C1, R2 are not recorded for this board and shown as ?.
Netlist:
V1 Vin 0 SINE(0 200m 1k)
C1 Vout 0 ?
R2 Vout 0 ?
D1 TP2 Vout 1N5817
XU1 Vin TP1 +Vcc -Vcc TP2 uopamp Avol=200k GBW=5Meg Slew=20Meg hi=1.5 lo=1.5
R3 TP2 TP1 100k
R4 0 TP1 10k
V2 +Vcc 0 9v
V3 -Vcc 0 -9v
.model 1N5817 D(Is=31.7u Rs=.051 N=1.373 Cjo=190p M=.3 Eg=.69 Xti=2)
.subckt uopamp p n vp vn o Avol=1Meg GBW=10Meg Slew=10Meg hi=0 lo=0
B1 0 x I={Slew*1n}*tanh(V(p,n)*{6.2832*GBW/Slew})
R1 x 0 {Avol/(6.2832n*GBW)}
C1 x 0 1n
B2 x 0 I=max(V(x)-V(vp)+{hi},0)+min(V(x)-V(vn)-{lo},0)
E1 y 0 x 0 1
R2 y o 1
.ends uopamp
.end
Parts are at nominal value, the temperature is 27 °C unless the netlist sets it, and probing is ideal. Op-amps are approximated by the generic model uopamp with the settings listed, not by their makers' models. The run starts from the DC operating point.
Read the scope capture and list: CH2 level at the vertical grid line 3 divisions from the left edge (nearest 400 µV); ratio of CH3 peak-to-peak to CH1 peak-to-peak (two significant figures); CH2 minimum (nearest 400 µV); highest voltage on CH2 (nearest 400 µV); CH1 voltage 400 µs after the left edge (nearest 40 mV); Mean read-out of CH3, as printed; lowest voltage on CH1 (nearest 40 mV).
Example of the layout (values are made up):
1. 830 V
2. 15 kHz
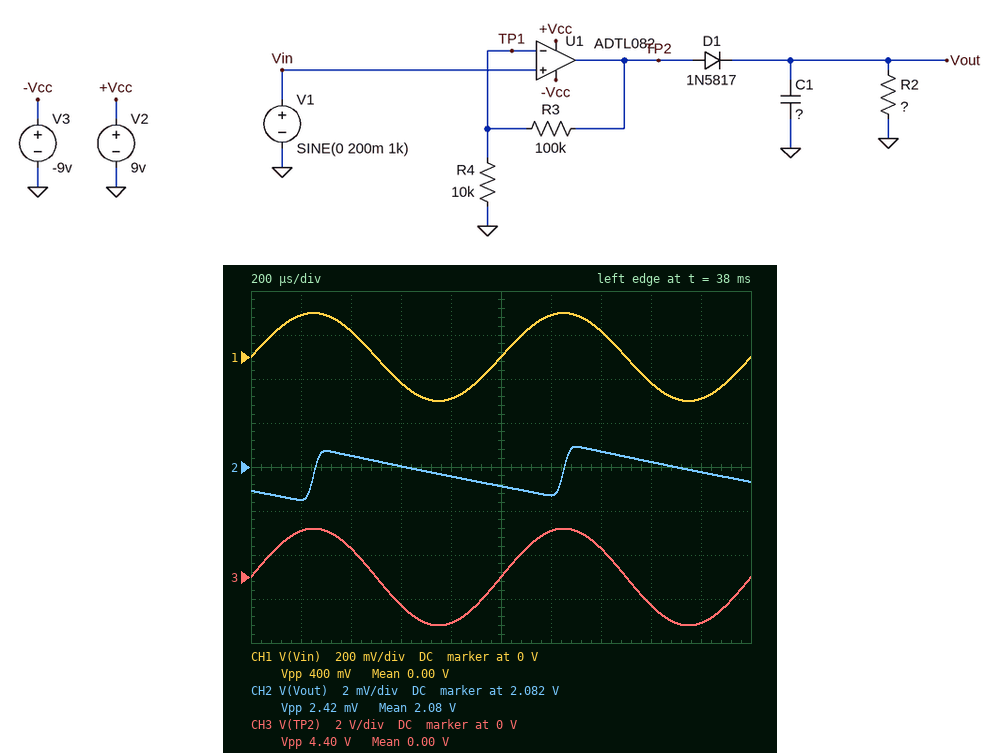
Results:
1. 2.0820 V
2. 11
3. 2.0804 V
4. 2.0828 V
5. 120 mV
6. 0.00 V
7. -200 mV
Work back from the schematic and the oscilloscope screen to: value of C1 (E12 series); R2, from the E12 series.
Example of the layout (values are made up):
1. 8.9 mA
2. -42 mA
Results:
1. 18 µF
2. 220 kΩ
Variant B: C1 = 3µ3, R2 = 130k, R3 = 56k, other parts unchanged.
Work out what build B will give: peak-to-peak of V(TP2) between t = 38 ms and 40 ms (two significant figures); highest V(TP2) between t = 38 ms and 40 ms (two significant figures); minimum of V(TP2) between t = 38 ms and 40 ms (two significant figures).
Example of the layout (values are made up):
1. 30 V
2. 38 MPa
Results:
1. 2.6 V
2. 1.3 V
3. -1.3 V
